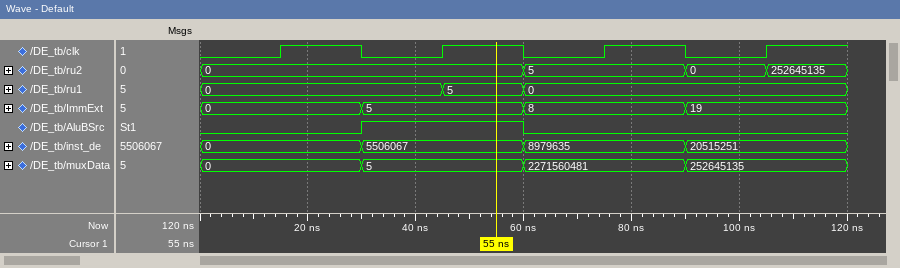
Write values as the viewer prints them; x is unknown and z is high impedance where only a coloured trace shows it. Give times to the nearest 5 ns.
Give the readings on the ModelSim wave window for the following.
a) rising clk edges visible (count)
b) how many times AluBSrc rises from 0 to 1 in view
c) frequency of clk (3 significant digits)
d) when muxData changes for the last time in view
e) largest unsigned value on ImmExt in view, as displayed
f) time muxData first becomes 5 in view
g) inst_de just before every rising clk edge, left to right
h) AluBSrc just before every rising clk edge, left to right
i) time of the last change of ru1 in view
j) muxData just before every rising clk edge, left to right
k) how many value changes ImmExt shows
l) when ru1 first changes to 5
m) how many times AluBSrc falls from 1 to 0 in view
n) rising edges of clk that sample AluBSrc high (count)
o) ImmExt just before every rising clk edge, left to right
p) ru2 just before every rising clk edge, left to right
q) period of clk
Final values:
4
1
33.3 MHz
90 ns
19
30 ns
0, 5506067, 8979635, 20515251
0 1 0 0
60 ns
0, 5, 2271560481, 252645135
3
45 ns
1
1
0, 5, 8, 19
0, 0, 5, 0
30 ns
